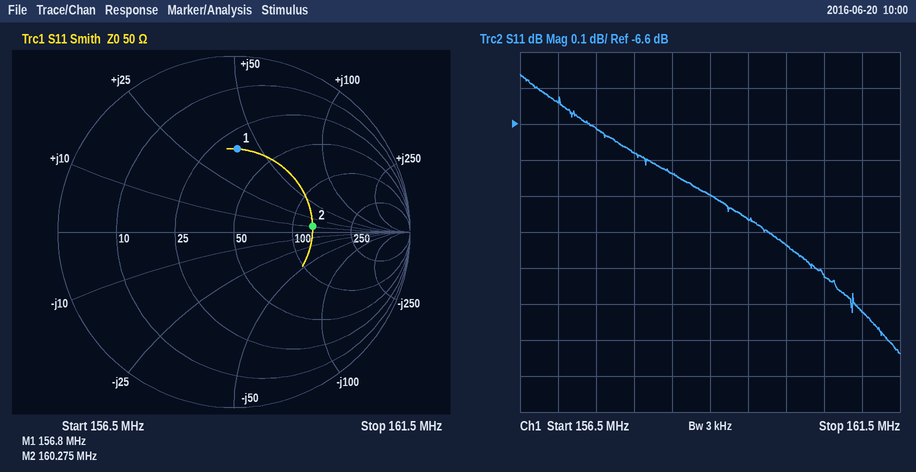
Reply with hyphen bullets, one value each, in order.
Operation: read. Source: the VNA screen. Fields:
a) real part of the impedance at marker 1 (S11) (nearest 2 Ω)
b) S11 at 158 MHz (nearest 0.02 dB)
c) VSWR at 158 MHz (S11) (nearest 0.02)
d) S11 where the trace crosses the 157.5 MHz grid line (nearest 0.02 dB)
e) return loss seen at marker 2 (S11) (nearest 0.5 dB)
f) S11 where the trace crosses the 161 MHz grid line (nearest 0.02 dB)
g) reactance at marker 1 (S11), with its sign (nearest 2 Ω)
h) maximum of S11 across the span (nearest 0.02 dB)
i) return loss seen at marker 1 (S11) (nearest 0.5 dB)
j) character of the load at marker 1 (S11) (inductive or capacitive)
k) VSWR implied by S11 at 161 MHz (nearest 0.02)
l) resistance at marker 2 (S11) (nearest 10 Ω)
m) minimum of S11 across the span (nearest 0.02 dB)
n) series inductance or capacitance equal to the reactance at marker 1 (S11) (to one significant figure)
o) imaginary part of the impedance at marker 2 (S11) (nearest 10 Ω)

- 32 Ω
- -6.68 dB
- 2.72
- -6.62 dB
- 7.0 dB
- -7.12 dB
- +40 Ω
- -6.46 dB
- 6.5 dB
- inductive
- 2.58
- 130 Ω
- -7.24 dB
- 40 nH
- +10 Ω
